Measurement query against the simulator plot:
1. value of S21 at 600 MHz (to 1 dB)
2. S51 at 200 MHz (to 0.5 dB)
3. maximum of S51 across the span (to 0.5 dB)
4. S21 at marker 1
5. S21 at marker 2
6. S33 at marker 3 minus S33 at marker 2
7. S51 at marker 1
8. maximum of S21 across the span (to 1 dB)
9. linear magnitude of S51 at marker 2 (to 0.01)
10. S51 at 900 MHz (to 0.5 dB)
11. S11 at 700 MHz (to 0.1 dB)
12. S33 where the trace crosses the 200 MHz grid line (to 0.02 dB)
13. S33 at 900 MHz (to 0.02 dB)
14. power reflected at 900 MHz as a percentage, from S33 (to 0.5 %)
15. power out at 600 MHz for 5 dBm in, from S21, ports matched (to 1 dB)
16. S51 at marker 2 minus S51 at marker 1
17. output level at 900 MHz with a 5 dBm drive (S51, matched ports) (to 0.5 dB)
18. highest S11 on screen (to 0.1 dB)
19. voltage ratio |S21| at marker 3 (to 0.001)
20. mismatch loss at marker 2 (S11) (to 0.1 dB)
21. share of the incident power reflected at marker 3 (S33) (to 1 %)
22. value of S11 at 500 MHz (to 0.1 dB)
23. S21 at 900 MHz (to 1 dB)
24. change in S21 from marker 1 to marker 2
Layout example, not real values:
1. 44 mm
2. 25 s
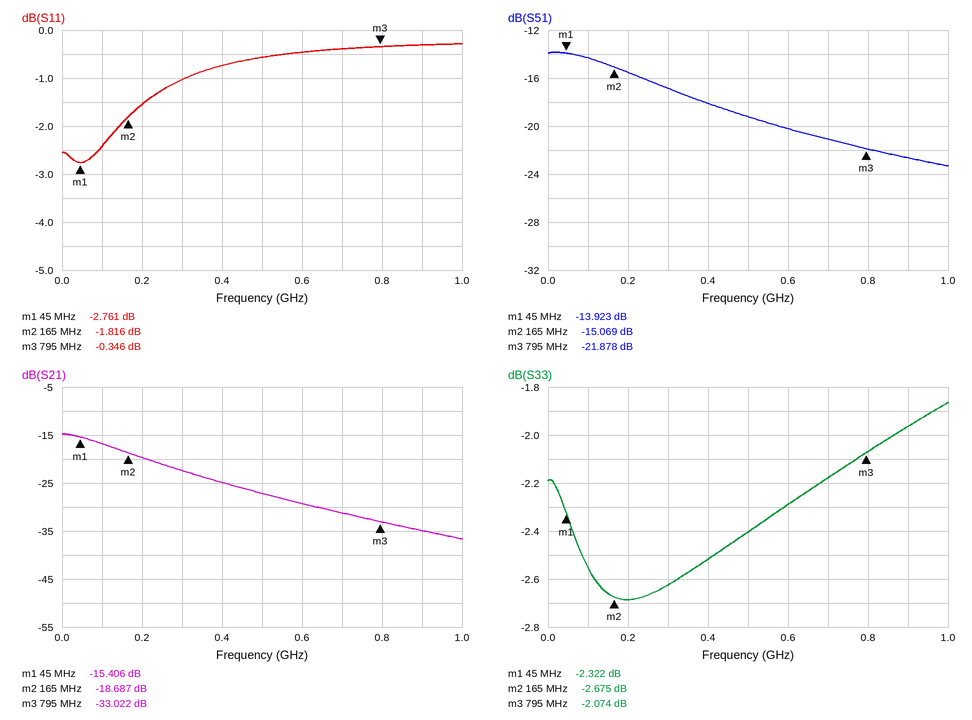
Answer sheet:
1. -29 dB
2. -15.5 dB
3. -14.0 dB
4. -15.406 dB
5. -18.687 dB
6. 0.601 dB
7. -13.923 dB
8. -15 dB
9. 0.18
10. -22.5 dB
11. -0.4 dB
12. -2.68 dB
13. -1.96 dB
14. 63.5 %
15. -24 dBm
16. -1.146 dB
17. -17.5 dBm
18. -0.3 dB
19. 0.022
20. 4.7 dB
21. 62 %
22. -0.6 dB
23. -35 dB
24. -3.281 dB
